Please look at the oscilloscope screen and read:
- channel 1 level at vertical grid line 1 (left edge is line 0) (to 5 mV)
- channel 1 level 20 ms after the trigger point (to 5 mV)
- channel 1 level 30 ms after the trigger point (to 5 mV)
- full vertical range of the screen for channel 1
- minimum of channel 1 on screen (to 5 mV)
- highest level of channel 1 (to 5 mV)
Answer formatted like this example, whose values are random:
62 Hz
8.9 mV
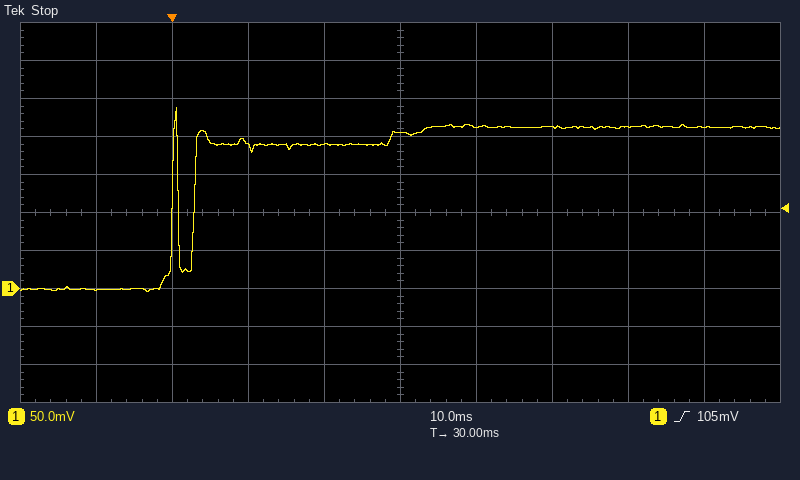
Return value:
0 mV
190 mV
205 mV
500 mV
-5 mV
240 mV
